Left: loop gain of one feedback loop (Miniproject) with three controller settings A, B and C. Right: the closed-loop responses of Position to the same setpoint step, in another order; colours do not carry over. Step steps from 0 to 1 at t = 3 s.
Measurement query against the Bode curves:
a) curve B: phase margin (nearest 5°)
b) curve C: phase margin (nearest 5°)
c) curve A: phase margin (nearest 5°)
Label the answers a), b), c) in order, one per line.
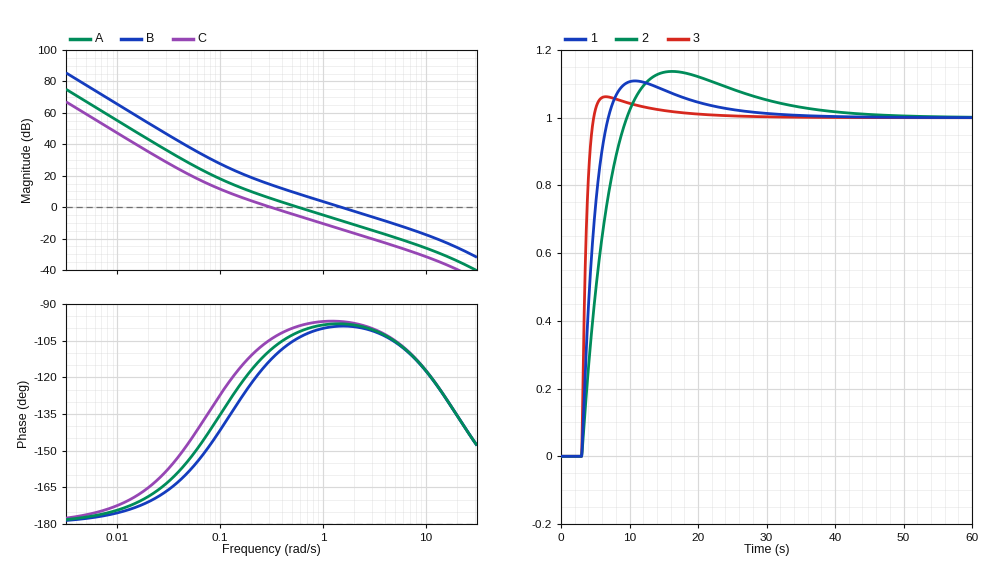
a) 80°
b) 75°
c) 80°
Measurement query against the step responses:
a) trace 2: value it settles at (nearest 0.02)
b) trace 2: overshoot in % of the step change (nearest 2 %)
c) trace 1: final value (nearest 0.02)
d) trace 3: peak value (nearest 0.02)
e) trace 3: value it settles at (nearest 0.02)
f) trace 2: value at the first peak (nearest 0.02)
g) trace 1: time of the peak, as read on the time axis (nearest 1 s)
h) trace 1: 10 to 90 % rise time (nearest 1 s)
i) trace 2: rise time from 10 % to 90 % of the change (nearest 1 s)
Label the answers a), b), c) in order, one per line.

a) 1.00
b) 14 %
c) 1.00
d) 1.06
e) 1.00
f) 1.14
g) 11 s
h) 3 s
i) 5 s
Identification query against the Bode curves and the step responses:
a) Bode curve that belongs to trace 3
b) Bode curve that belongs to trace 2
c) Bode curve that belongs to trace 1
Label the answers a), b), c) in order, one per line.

a) B
b) C
c) A
